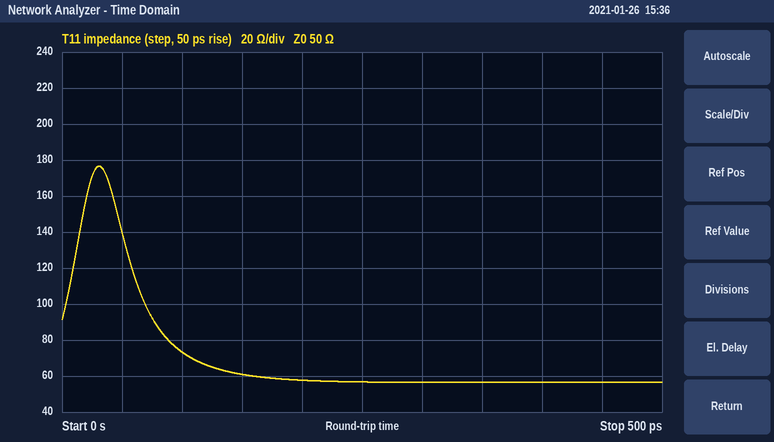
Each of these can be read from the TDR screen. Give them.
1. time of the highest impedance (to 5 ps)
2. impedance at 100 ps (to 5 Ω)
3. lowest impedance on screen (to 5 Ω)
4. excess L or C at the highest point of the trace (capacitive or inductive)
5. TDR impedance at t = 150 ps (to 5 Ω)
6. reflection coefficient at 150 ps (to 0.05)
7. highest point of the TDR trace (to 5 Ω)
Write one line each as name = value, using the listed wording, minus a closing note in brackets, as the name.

time of the highest impedance = 30 ps
impedance at 100 ps = 75 Ω
lowest impedance on screen = 55 Ω
excess L or C at the highest point of the trace = inductive
TDR impedance at t = 150 ps = 60 Ω
reflection coefficient at 150 ps = +0.10
highest point of the TDR trace = 175 Ω
